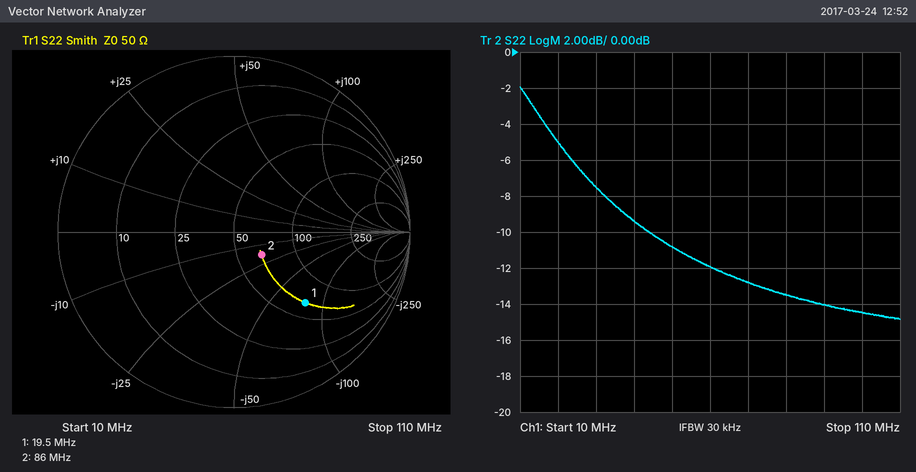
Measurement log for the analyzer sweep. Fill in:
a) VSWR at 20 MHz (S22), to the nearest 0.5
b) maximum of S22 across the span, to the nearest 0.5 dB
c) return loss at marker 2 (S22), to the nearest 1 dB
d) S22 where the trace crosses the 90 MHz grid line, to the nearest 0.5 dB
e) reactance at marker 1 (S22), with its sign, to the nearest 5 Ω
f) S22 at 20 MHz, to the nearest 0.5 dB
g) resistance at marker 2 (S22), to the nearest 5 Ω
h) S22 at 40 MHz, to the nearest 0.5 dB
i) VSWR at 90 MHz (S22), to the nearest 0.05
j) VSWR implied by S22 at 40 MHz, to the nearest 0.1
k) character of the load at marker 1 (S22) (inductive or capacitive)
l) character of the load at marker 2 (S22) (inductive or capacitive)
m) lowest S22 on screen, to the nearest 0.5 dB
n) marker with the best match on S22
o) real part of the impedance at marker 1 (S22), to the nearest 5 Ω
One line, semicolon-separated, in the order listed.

3.5; -2.0 dB; 14 dB; -14.0 dB; -80 Ω; -5.0 dB; 65 Ω; -9.5 dB; 1.50; 2.0; capacitive; capacitive; -15.0 dB; marker 2; 65 Ω
